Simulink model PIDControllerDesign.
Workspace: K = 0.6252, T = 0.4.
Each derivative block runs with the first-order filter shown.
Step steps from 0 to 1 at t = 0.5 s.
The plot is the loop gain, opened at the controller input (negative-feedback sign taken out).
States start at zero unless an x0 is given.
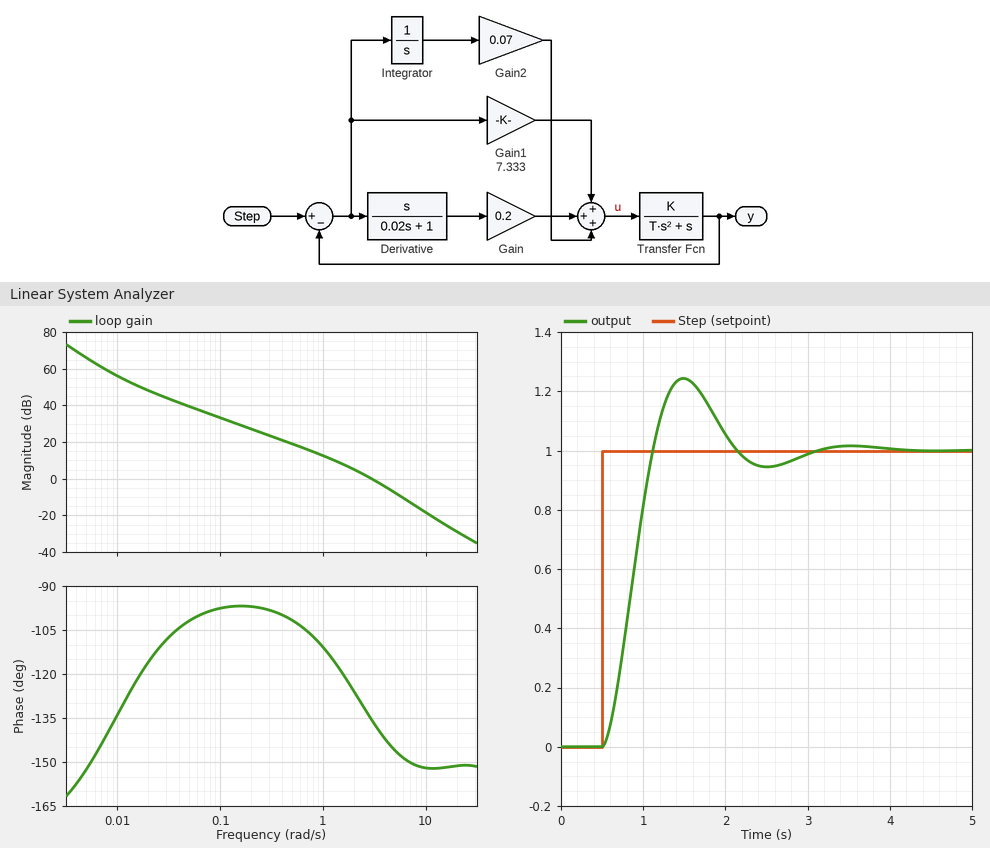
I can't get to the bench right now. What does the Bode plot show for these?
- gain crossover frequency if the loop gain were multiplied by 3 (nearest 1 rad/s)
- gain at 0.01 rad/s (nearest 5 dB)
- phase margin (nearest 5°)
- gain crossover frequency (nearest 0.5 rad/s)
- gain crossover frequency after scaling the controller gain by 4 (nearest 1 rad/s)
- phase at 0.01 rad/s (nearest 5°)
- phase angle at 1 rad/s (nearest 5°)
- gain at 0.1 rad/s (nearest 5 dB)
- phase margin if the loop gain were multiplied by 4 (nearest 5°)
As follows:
6 rad/s
55 dB
45°
3.0 rad/s
7 rad/s
-135°
-110°
35 dB
30°
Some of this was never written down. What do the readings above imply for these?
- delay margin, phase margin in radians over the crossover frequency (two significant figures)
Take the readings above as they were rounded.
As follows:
0.26 s
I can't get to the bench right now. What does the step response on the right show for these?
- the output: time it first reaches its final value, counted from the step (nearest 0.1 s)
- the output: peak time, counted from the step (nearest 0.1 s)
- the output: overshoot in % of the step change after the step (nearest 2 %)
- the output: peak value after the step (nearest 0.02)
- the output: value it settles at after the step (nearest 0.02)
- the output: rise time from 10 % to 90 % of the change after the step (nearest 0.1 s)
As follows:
0.6 s
1.0 s
24 %
1.24
1.00
0.4 s
